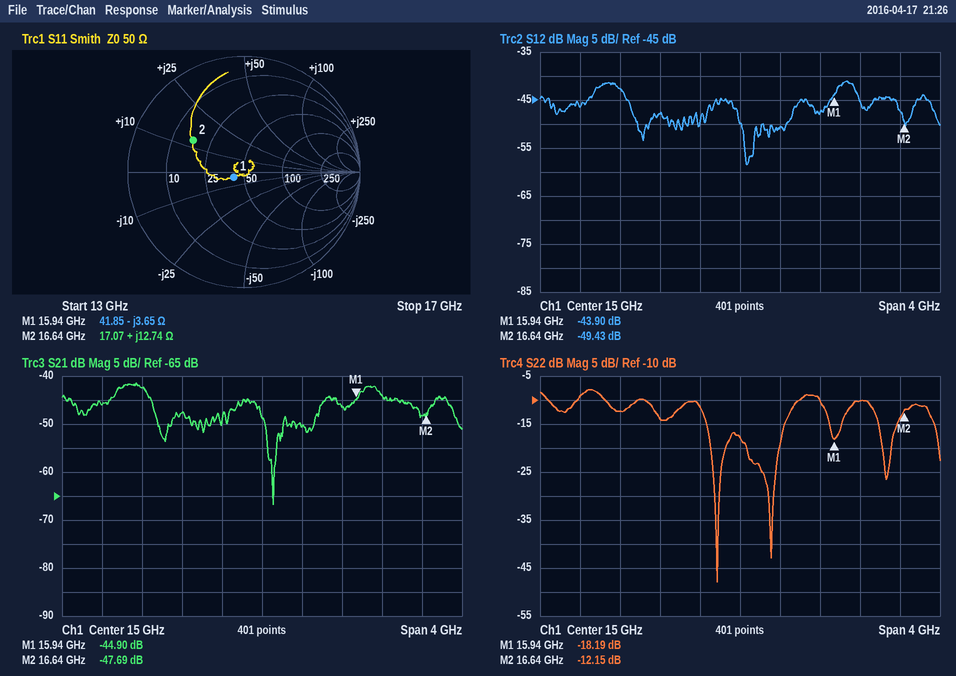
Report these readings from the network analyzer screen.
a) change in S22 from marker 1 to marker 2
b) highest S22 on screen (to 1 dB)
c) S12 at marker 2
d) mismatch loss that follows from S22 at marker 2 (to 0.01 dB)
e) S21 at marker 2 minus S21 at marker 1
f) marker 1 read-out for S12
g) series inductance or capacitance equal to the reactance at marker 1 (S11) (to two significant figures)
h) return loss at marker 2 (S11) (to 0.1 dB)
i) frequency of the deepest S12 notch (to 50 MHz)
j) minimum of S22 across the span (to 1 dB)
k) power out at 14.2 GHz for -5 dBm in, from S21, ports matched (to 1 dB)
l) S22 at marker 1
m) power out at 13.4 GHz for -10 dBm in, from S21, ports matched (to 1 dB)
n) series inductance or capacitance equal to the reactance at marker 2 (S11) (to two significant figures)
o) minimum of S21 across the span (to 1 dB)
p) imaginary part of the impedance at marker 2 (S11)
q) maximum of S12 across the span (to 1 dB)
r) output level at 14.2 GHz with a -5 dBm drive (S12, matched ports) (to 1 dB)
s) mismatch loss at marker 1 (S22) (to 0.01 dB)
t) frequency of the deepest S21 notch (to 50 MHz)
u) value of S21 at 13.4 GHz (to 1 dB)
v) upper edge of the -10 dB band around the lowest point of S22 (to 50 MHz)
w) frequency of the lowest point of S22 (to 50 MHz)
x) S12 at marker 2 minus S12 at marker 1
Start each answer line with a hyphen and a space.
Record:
- 6.04 dB
- -8 dB
- -49.43 dB
- 0.27 dB
- -2.79 dB
- -43.90 dB
- 2.7 pF
- 5.7 dB
- 15.05 GHz
- -48 dB
- -53 dBm
- -18.19 dB
- -56 dBm
- 120 pH
- -67 dB
- +12.74 Ω
- -41 dB
- -53 dBm
- 0.07 dB
- 15.10 GHz
- -46 dB
- 15.60 GHz
- 14.75 GHz
- -5.53 dB
